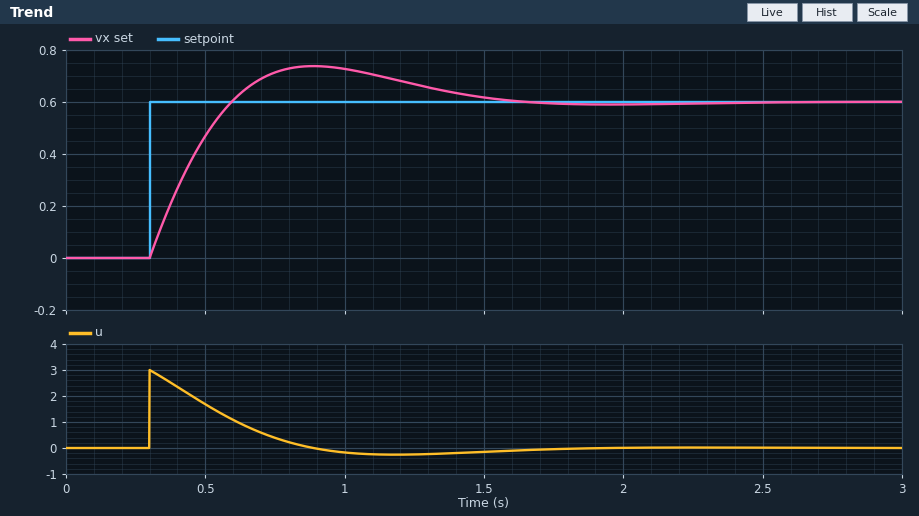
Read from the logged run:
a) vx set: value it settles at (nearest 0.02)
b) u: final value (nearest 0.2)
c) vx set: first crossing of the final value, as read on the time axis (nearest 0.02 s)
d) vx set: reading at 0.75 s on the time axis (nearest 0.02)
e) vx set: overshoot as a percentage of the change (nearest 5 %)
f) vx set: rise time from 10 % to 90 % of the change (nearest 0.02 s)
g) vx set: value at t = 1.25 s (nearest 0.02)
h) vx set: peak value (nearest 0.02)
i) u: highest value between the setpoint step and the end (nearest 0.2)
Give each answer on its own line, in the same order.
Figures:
0.60
0.0
0.60 s
0.72
25 %
0.22 s
0.66
0.74
3.0
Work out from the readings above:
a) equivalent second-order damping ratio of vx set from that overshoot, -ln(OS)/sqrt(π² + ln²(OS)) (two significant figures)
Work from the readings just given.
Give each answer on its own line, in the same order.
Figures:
0.40
